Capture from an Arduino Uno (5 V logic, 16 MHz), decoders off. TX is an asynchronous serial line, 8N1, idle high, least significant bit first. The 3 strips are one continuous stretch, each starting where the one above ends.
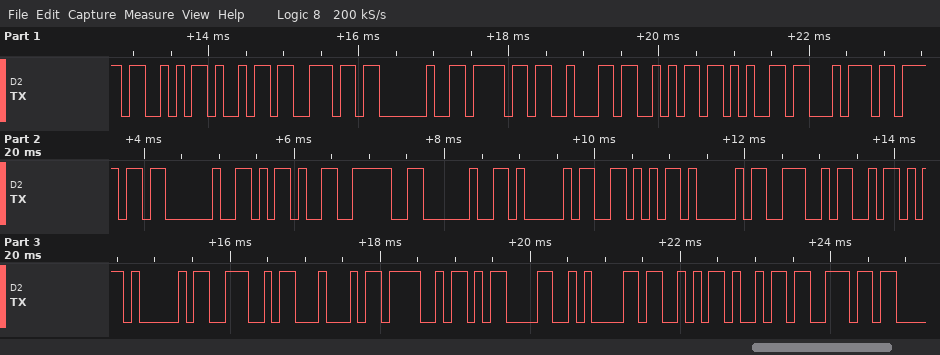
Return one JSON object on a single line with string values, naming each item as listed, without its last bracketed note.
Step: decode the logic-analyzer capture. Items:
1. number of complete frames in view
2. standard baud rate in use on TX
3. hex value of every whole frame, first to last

{"number of complete frames in view": "28", "standard baud rate in use on TX": "9600 baud", "hex value of every whole frame, first to last": "0x53 0x69 0x6E 0x20 0x6F 0x62 0x6A 0x65 0x74 0x6F 0x20 0x2D 0x3E 0x20 0x41 0x56 0x41 0x4E 0x5A 0x41 0x4E 0x44 0x4F 0x0D 0x0A 0x53 0x69 0x6E"}
